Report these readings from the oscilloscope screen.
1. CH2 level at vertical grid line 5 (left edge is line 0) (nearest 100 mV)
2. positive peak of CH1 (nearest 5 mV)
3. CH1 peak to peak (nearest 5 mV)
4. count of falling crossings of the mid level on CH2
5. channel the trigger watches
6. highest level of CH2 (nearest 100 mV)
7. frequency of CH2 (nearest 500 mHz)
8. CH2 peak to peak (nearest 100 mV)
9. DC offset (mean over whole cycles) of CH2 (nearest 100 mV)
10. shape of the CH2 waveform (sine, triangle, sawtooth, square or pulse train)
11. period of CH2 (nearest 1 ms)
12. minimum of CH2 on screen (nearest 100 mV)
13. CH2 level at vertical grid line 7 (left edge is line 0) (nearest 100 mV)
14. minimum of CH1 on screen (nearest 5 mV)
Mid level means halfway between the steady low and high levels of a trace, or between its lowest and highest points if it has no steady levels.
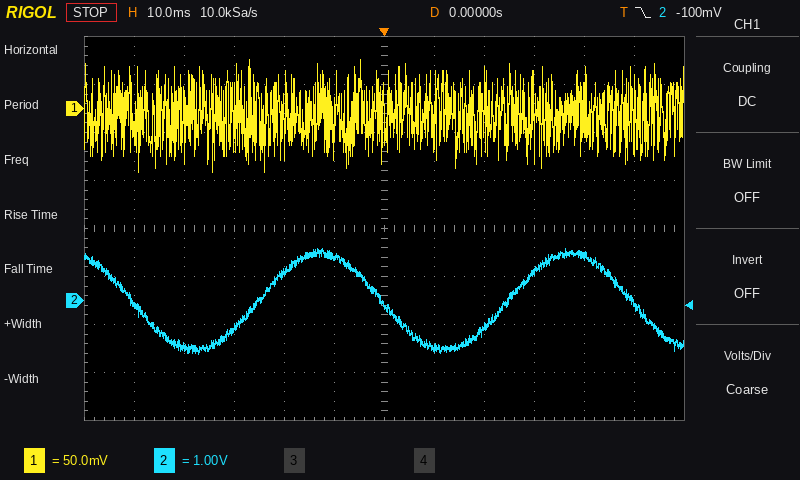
900 mV
50 mV
115 mV
3
CH2
1.1 V
20.0 Hz
2.2 V
0.0 V
sine
50 ms
-1.1 V
-1.0 V
-65 mV
